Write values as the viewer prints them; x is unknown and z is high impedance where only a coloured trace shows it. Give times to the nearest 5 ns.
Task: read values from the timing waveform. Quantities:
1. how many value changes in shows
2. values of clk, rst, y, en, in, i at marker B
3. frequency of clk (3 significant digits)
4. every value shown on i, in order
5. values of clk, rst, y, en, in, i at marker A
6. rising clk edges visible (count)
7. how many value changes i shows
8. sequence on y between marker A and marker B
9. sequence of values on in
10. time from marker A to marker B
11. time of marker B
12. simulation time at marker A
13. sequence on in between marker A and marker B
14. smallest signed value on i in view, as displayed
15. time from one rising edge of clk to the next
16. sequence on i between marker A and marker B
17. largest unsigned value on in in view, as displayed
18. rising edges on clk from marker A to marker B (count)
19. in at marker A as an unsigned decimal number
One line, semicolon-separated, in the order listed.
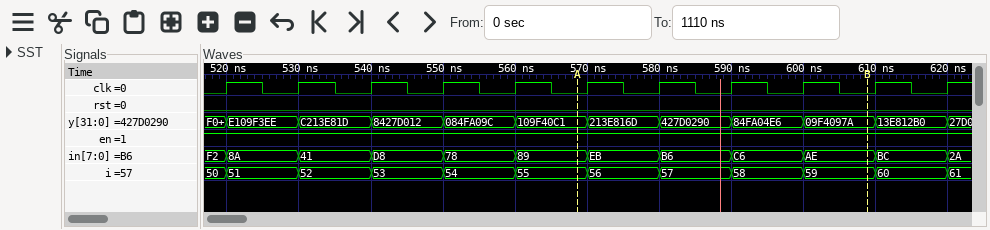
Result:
11; clk=0, rst=0, y=09F4097A, en=1, in=AE, i=59; 100 MHz; 50, 51, 52, 53, 54, 55, 56, 57, 58, 59, 60, 61; clk=0, rst=0, y=109F40C1, en=1, in=89, i=55; 11; 11; 109F40C1, 213E816D, 427D0290, 84FA04E6, 09F4097A; F2, 8A, 41, D8, 78, 89, EB, B6, C6, AE, BC, 2A; 40 ns; 610 ns; 570 ns; 89, EB, B6, C6, AE; 50; 10 ns; 55, 56, 57, 58, 59; F2; 4; 137
